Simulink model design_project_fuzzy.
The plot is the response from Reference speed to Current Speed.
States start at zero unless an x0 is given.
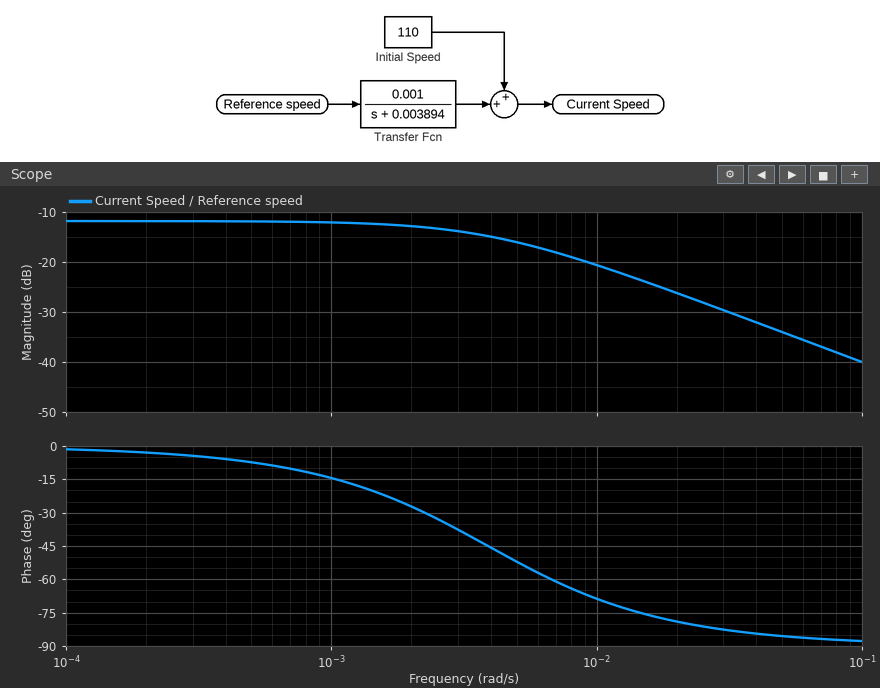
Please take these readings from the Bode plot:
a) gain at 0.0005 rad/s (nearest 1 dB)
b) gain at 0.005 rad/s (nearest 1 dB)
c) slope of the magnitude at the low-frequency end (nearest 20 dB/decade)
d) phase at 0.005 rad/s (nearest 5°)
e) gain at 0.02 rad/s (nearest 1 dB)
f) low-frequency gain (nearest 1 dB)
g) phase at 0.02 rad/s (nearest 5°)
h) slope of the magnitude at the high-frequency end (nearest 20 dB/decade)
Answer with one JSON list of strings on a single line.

["-12 dB", "-16 dB", "0 dB/decade", "-50°", "-26 dB", "-12 dB", "-80°", "-20 dB/decade"]
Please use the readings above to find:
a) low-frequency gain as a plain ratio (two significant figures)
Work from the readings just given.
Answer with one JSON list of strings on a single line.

["0.25"]
